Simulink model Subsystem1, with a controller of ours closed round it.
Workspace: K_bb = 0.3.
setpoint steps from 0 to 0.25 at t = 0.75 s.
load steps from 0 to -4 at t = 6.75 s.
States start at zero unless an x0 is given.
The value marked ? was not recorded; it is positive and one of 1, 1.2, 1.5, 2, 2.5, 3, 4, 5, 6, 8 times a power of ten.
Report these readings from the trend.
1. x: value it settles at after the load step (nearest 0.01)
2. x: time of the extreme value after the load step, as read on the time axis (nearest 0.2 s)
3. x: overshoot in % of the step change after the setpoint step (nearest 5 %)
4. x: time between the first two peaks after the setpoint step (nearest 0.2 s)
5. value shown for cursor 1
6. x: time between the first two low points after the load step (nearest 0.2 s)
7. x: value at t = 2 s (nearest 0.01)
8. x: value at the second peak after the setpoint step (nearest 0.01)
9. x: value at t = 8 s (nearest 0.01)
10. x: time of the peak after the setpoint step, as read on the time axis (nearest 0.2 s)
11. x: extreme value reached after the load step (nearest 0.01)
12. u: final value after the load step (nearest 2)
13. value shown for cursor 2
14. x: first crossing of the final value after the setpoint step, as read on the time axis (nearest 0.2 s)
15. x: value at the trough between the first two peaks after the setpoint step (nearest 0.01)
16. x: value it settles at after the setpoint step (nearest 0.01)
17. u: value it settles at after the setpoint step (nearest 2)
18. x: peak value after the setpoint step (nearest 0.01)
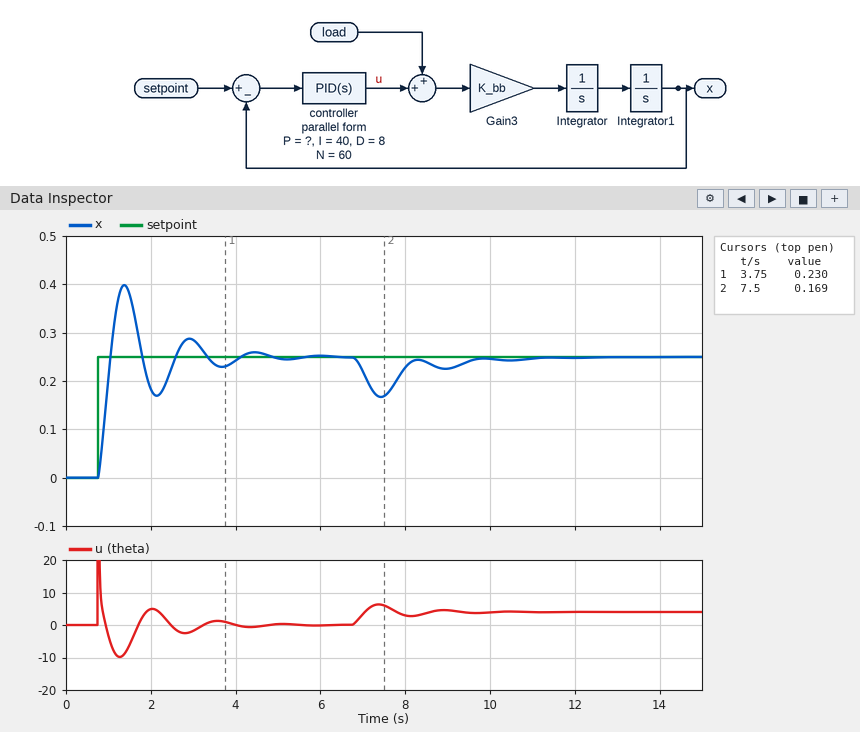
0.25
7.4 s
60 %
1.6 s
0.230
1.6 s
0.18
0.29
0.23
1.4 s
0.17
4
0.169
1.0 s
0.17
0.25
0
0.40
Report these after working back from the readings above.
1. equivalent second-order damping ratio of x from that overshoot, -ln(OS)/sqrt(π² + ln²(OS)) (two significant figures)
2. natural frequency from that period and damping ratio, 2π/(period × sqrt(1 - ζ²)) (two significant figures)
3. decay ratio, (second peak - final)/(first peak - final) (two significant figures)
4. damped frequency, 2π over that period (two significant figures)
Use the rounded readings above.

0.16
4.0 rad/s
0.27
3.9 rad/s
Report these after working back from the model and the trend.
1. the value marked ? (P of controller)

60
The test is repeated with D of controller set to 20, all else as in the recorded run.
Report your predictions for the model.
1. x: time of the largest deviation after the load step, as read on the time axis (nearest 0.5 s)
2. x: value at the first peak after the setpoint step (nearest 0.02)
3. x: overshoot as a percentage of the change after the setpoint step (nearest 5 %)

7.5 s
0.32
25 %
